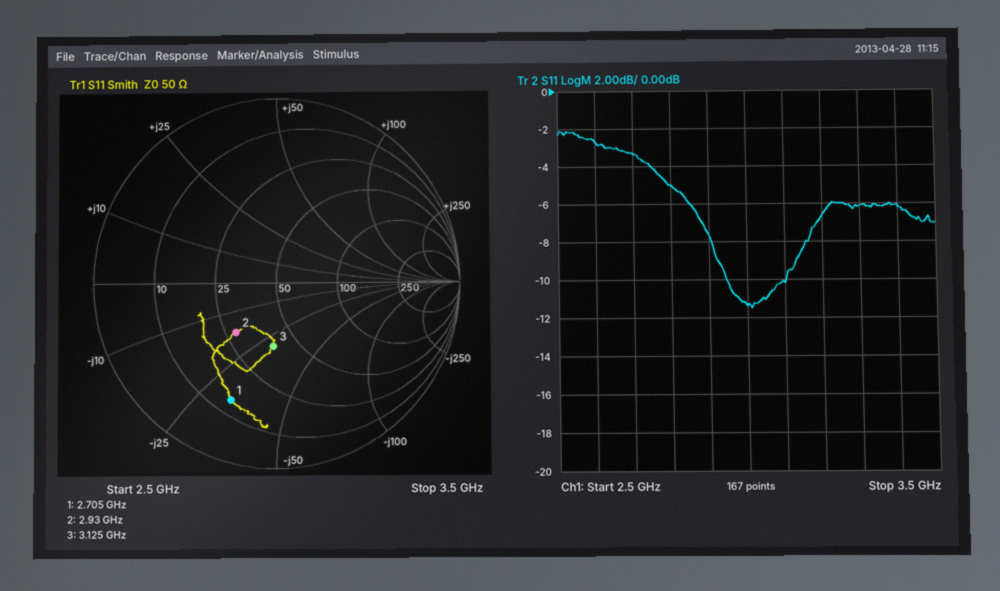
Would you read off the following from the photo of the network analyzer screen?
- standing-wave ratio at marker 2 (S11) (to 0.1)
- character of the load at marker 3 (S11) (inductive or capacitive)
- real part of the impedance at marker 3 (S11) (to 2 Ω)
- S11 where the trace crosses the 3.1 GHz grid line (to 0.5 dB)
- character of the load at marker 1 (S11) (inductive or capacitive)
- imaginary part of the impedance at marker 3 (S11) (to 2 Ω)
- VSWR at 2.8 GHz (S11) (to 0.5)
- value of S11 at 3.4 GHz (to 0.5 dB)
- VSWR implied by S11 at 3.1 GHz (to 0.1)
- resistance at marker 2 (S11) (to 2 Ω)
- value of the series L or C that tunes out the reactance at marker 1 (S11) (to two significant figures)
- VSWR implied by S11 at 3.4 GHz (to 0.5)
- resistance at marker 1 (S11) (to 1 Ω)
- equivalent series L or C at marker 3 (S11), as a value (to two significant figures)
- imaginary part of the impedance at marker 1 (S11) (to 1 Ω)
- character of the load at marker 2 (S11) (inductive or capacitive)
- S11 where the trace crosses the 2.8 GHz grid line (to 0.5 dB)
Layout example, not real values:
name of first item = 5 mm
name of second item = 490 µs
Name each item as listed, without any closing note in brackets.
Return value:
standing-wave ratio at marker 2 (S11) = 2.1
character of the load at marker 3 (S11) = capacitive
real part of the impedance at marker 3 (S11) = 38 Ω
S11 where the trace crosses the 3.1 GHz grid line = -10.0 dB
character of the load at marker 1 (S11) = capacitive
imaginary part of the impedance at marker 3 (S11) = -30 Ω
VSWR at 2.8 GHz (S11) = 3.5
value of S11 at 3.4 GHz = -6.0 dB
VSWR implied by S11 at 3.1 GHz = 1.9
resistance at marker 2 (S11) = 28 Ω
value of the series L or C that tunes out the reactance at marker 1 (S11) = 1.9 nH
VSWR implied by S11 at 3.4 GHz = 3.0
resistance at marker 1 (S11) = 14 Ω
equivalent series L or C at marker 3 (S11), as a value = 1.7 pF
imaginary part of the impedance at marker 1 (S11) = -32 Ω
character of the load at marker 2 (S11) = capacitive
S11 where the trace crosses the 2.8 GHz grid line = -5.0 dB
